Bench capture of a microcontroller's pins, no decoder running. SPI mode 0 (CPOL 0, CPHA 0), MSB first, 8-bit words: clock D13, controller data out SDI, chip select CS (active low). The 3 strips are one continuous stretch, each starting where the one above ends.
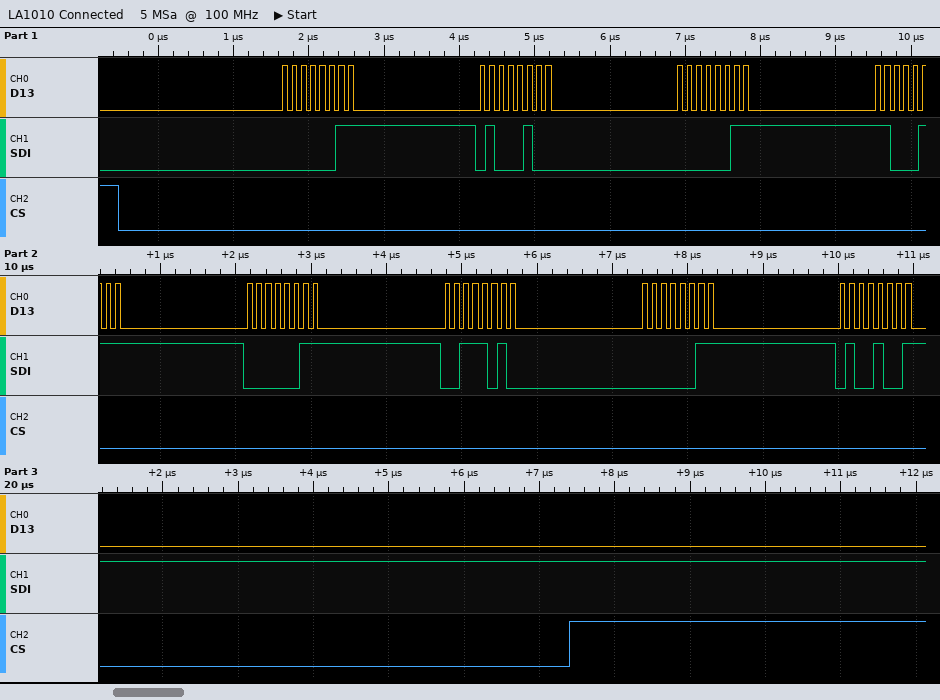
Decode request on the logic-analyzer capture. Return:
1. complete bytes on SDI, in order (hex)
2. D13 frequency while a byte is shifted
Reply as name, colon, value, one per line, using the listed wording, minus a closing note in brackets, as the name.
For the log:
complete bytes on SDI, in order: 03 44 03 C7 03 3A 03 49
D13 frequency while a byte is shifted: 8 MHz
